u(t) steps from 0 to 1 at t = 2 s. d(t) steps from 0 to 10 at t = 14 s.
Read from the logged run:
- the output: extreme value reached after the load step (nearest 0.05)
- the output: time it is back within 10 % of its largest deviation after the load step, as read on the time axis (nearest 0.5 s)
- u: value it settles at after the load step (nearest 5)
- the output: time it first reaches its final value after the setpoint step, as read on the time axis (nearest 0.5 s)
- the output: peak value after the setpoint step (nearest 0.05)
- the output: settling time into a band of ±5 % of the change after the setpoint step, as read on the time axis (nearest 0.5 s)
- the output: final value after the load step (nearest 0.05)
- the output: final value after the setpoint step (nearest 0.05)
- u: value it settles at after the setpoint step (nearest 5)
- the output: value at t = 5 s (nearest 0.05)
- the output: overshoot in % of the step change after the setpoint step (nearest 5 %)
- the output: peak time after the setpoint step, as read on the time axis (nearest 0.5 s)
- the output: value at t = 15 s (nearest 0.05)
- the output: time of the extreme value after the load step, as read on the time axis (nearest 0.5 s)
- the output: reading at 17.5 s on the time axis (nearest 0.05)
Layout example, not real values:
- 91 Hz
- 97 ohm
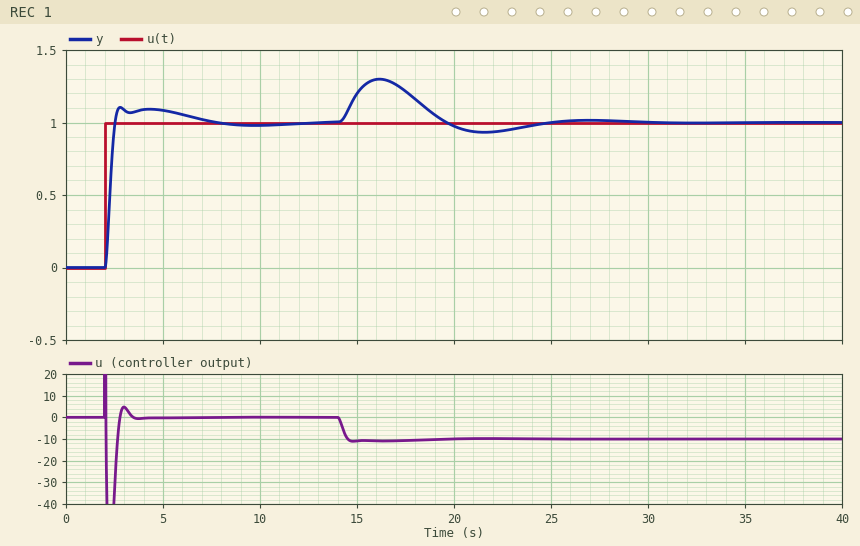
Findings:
- 1.30
- 23.5 s
- -10
- 2.5 s
- 1.10
- 6.0 s
- 1.00
- 1.00
- 0
- 1.10
- 10 %
- 3.0 s
- 1.20
- 16.0 s
- 1.20
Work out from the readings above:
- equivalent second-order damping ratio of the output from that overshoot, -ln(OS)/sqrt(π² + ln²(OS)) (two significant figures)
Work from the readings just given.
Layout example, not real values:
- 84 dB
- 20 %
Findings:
- 0.59
